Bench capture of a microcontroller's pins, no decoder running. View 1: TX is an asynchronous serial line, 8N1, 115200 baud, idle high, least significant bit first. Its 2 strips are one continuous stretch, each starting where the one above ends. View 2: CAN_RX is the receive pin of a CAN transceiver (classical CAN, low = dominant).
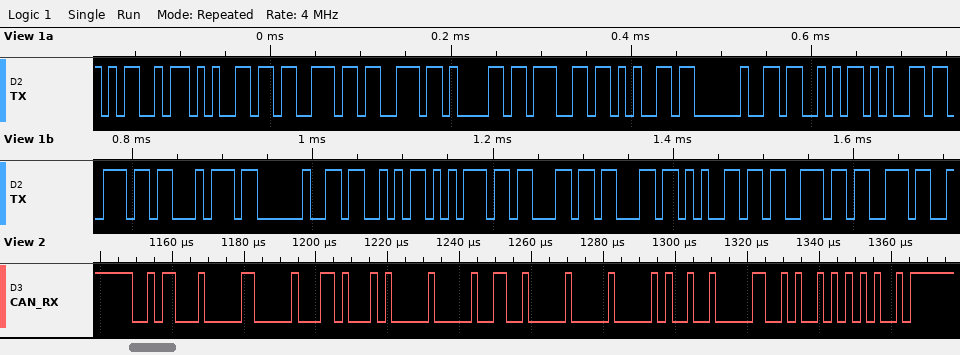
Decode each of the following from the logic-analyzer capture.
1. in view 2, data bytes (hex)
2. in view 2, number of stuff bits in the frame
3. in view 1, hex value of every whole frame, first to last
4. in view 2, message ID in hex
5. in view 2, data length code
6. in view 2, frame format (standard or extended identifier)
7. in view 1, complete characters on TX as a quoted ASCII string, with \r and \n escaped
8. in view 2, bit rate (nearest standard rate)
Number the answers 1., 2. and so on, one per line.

1. 06 8A 00 19 00 00 92 09
2. 8
3. 4D 65 73 73 61 67 65 20 53 65 6E 74 20 53 75 63 63 65 73 73
4. 0x2C4
5. 8
6. standard
7. "Message Sent Success"
8. 500 kbit/s
